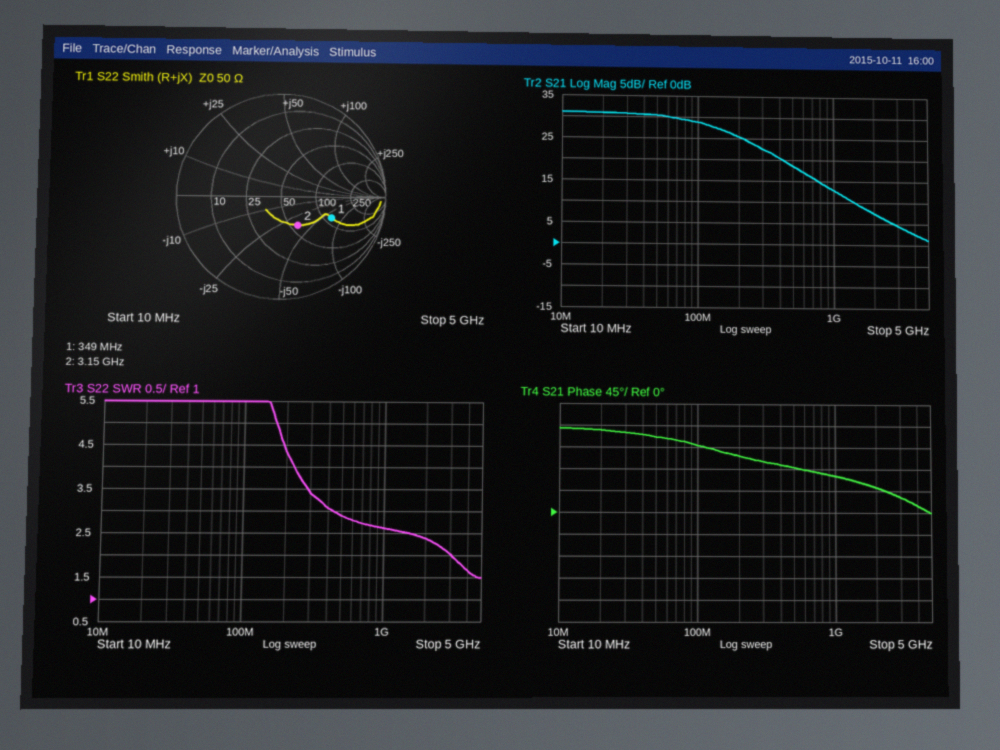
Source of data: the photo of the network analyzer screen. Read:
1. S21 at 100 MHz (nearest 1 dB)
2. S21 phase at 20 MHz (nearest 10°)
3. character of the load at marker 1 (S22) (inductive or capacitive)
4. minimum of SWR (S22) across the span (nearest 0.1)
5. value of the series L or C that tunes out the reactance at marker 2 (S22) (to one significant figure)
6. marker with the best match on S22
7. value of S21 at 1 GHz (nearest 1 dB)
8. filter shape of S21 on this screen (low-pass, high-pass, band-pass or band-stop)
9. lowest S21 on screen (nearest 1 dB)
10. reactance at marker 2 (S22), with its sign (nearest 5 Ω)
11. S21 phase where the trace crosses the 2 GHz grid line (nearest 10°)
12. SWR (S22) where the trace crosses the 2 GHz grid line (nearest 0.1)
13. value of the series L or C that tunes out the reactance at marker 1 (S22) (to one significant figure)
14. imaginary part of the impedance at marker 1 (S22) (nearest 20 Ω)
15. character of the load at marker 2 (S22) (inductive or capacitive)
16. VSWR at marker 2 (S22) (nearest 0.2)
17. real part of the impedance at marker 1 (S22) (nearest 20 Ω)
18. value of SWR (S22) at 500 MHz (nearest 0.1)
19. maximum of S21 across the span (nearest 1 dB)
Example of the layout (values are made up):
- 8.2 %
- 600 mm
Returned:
- 29 dB
- 170°
- capacitive
- 1.5
- 2 nH
- marker 2
- 13 dB
- low-pass
- 1 dB
- -35 Ω
- 50°
- 2.4
- 30 nH
- -60 Ω
- capacitive
- 2.0
- 120 Ω
- 2.9
- 31 dB
